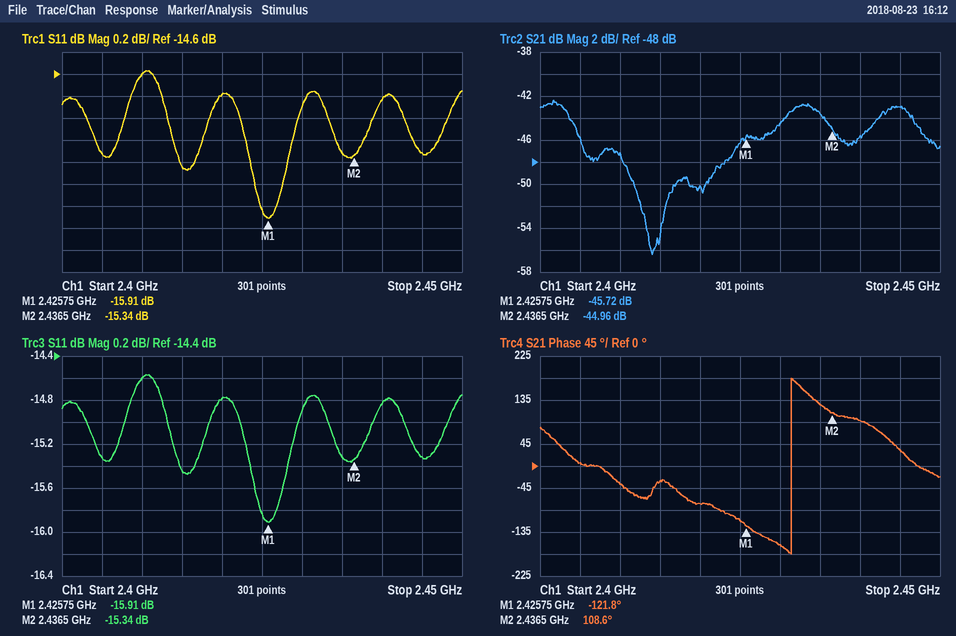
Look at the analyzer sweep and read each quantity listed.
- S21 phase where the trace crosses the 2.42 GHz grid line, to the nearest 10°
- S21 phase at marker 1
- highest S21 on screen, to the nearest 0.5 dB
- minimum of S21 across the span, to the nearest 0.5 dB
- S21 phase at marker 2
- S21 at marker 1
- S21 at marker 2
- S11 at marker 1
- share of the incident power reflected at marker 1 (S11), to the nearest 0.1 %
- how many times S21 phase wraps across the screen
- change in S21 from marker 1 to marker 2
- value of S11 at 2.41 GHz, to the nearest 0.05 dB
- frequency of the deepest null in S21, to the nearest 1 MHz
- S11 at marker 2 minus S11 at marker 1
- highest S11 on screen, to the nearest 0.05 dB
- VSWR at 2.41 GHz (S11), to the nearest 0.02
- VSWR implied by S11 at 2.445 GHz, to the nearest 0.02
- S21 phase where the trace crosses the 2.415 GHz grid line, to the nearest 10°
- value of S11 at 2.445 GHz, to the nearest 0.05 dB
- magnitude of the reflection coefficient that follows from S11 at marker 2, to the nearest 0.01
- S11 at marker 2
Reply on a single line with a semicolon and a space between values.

-80°; -121.8°; -42.5 dB; -56.5 dB; 108.6°; -45.72 dB; -44.96 dB; -15.91 dB; 2.6 %; 1; 0.76 dB; -14.60 dB; 2.414 GHz; 0.57 dB; -14.55 dB; 1.46; 1.42; -30°; -15.30 dB; 0.17; -15.34 dB
